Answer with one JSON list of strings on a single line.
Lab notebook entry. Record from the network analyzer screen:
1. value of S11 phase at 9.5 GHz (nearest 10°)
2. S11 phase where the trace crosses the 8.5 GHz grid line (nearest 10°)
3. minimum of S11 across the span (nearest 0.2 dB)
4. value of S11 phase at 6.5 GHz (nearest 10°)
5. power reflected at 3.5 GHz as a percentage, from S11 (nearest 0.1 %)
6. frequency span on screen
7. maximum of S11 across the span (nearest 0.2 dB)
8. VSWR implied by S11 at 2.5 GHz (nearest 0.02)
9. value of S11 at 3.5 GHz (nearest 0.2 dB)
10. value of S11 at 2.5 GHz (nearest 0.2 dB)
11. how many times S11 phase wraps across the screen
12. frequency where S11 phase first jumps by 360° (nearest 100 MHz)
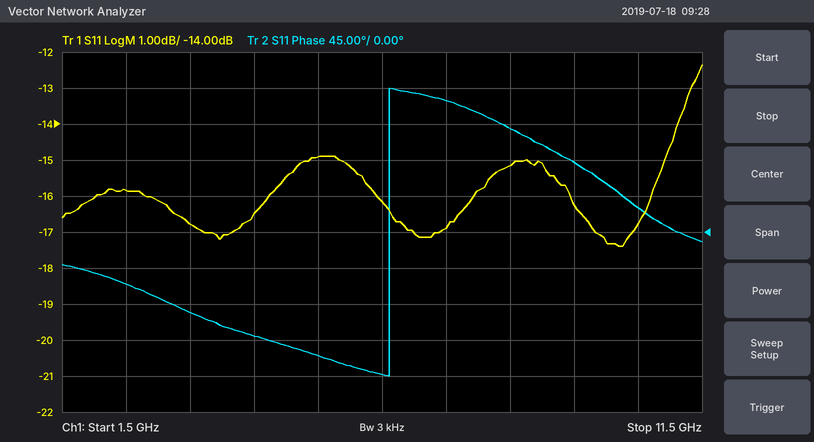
["90°", "130°", "-17.4 dB", "-180°", "2.1 %", "10 GHz", "-12.4 dB", "1.38", "-16.8 dB", "-15.8 dB", "1", "6.6 GHz"]
